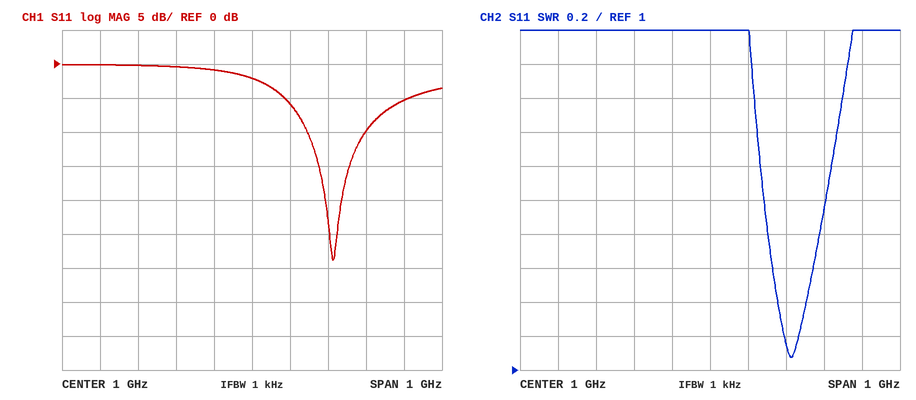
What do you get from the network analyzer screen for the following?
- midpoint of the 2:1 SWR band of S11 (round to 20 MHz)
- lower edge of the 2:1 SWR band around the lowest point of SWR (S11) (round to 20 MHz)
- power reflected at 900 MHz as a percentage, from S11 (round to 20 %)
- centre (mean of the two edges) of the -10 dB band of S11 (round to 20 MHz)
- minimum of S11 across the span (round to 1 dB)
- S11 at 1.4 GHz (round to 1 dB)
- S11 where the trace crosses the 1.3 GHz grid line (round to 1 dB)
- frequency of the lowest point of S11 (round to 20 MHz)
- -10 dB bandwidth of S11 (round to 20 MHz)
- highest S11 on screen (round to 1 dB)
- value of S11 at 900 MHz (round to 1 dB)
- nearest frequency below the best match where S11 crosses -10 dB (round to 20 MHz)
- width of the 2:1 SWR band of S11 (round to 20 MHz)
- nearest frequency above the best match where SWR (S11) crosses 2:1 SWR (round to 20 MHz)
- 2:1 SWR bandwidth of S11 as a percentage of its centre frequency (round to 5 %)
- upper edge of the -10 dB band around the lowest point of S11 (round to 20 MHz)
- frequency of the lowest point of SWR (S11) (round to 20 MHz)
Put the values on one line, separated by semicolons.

1.22 GHz; 1.14 GHz; 80 %; 1.22 GHz; -29 dB; -5 dB; -10 dB; 1.22 GHz; 160 MHz; 0 dB; -1 dB; 1.14 GHz; 160 MHz; 1.30 GHz; 15 %; 1.30 GHz; 1.22 GHz
